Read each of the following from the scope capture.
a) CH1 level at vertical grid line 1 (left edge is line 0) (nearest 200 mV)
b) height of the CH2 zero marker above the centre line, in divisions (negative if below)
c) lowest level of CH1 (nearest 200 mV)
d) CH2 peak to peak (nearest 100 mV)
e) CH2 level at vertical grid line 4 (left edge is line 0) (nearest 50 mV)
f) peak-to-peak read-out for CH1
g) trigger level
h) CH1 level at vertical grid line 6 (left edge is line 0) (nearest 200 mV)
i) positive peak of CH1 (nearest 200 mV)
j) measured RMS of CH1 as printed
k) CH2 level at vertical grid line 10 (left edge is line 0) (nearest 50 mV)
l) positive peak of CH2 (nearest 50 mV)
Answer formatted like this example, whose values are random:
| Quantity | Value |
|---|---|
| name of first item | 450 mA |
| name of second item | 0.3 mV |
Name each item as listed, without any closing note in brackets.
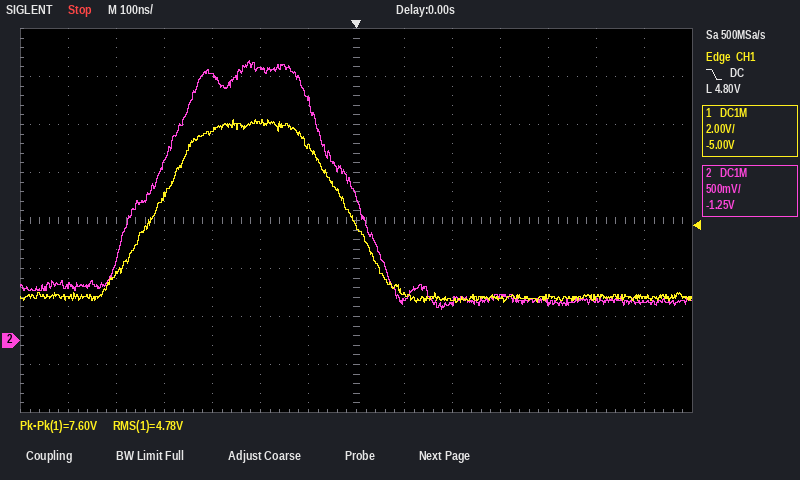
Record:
| Quantity | Value |
|---|---|
| CH1 level at vertical grid line 1 (left edge is line 0) | 1.8 V |
| height of the CH2 zero marker above the centre line, in divisions | -2.5 div |
| lowest level of CH1 | 1.6 V |
| CH2 peak to peak | 2.60 V |
| CH2 level at vertical grid line 4 (left edge is line 0) | 2.75 V |
| peak-to-peak read-out for CH1 | 7.60 V |
| trigger level | 4.80 V |
| CH1 level at vertical grid line 6 (left edge is line 0) | 8.0 V |
| positive peak of CH1 | 9.2 V |
| measured RMS of CH1 as printed | 4.78 V |
| CH2 level at vertical grid line 10 (left edge is line 0) | 450 mV |
| positive peak of CH2 | 2.90 V |
